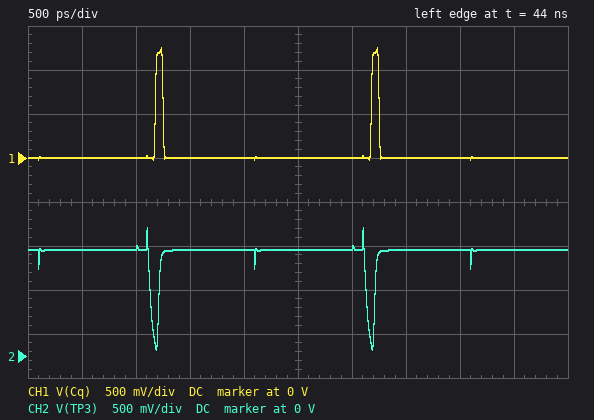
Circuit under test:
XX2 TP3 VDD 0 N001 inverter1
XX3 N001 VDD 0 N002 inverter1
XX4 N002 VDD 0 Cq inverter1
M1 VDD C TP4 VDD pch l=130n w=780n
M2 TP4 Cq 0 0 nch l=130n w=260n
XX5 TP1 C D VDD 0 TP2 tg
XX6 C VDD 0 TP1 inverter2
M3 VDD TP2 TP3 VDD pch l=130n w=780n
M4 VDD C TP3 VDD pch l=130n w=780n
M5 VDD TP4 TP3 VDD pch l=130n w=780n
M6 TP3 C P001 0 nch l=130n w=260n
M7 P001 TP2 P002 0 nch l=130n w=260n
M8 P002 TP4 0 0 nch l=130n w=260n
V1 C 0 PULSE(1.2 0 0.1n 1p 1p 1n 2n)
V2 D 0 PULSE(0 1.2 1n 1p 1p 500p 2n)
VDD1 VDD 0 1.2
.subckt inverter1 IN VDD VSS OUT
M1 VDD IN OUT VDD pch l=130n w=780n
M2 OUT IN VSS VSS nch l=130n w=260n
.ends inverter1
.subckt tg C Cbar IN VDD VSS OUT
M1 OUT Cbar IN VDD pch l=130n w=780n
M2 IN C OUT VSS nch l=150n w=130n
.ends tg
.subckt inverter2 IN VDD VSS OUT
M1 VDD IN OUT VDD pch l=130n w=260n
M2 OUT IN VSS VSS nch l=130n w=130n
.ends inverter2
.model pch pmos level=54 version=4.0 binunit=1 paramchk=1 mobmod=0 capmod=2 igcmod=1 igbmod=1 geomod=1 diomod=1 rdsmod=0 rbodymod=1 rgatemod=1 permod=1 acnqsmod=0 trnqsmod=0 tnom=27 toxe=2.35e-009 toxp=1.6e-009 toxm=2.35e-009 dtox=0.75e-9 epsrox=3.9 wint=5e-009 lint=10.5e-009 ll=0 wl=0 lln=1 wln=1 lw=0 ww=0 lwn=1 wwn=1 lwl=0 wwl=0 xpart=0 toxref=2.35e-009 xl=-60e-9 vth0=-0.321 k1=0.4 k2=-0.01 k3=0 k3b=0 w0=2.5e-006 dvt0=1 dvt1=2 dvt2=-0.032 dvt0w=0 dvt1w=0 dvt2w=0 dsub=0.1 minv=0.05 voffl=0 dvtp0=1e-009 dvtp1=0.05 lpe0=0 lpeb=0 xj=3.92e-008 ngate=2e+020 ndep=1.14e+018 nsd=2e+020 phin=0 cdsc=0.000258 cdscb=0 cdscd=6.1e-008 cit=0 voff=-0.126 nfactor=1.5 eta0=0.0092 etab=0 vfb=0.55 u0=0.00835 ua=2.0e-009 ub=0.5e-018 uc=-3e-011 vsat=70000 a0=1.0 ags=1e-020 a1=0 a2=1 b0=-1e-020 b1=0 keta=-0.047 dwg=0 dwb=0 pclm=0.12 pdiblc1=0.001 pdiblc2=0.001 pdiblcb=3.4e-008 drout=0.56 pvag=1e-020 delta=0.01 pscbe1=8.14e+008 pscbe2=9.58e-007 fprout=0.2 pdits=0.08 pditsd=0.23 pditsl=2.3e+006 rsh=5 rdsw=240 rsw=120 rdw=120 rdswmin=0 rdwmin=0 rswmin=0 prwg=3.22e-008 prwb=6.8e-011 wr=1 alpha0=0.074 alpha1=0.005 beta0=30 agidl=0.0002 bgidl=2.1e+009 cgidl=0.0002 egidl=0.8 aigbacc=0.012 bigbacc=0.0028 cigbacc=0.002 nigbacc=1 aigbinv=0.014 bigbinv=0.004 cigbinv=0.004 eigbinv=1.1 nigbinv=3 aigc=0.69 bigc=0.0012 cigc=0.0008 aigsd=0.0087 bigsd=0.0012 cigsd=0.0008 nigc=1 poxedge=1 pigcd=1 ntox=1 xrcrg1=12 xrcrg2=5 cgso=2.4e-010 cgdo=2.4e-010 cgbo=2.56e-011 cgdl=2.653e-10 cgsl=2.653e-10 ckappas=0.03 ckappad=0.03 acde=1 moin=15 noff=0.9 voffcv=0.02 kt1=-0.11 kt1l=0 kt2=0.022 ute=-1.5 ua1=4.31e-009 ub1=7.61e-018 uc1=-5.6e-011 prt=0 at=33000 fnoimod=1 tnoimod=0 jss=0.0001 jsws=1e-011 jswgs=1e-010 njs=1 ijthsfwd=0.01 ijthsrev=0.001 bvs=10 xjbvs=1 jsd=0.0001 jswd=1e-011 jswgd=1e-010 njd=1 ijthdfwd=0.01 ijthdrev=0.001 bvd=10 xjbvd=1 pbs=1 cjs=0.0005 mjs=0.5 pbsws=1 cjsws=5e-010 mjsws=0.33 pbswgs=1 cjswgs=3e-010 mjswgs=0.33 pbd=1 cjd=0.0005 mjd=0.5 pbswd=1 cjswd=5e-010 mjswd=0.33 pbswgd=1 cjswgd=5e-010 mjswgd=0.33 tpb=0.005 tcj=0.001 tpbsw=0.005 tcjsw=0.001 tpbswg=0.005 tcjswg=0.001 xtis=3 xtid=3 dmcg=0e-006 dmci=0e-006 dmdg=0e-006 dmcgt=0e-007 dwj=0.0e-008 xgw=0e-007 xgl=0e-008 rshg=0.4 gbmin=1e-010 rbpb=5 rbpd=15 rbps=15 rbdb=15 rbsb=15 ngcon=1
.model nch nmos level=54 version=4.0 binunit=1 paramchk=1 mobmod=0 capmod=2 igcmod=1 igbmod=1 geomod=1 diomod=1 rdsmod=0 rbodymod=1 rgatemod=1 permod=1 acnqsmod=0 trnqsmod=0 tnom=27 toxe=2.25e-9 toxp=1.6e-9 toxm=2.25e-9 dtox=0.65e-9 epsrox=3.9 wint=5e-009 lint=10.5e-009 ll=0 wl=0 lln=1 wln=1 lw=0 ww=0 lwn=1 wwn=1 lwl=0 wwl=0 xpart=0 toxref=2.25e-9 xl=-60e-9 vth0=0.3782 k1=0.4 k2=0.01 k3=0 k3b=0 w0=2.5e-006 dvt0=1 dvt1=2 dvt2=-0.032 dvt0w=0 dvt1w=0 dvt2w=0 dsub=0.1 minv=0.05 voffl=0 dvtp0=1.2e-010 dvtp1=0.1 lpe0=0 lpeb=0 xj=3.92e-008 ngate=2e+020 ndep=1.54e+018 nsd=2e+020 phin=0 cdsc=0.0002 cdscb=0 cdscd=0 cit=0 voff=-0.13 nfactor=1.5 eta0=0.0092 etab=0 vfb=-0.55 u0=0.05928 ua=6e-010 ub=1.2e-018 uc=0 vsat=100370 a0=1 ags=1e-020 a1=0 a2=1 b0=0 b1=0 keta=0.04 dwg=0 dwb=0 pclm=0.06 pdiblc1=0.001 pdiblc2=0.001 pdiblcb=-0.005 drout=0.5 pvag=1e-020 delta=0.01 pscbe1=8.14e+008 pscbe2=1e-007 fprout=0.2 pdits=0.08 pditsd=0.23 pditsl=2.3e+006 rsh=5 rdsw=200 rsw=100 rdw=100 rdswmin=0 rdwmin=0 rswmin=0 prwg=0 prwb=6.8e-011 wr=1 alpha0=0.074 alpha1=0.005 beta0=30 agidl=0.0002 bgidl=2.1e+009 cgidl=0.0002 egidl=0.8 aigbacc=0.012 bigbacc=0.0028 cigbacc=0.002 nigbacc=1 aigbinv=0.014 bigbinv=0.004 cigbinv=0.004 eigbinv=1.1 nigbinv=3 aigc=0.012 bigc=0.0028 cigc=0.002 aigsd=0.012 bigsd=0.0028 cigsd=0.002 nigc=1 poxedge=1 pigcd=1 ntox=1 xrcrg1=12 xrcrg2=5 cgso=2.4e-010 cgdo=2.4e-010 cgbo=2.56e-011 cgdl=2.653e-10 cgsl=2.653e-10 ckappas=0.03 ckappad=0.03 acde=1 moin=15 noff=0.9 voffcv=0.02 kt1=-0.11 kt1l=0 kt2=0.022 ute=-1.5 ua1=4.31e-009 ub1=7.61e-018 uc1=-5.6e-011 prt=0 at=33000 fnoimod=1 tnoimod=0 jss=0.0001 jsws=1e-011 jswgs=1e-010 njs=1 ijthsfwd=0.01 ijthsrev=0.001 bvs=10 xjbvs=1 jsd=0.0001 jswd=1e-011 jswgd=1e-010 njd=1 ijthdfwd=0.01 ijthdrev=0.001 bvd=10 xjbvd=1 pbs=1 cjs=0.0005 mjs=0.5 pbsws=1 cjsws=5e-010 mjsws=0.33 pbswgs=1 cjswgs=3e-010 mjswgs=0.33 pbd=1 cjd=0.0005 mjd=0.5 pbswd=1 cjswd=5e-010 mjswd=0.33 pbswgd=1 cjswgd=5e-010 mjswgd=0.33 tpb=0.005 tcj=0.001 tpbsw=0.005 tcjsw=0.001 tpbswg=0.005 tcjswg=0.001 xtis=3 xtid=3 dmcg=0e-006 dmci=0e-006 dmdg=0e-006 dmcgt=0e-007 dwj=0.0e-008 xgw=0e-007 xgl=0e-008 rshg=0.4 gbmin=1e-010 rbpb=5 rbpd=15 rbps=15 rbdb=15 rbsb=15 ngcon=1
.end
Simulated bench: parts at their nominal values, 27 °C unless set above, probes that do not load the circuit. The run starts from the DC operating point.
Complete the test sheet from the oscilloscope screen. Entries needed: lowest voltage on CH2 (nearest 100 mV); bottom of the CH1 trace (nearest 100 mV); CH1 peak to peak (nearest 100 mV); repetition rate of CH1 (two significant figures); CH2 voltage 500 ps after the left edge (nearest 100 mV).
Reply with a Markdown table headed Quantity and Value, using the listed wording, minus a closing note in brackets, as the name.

| Quantity | Value |
|---|---|
| lowest voltage on CH2 | 100 mV |
| bottom of the CH1 trace | 0 V |
| CH1 peak to peak | 1.3 V |
| repetition rate of CH1 | 500 MHz |
| CH2 voltage 500 ps after the left edge | 1.2 V |
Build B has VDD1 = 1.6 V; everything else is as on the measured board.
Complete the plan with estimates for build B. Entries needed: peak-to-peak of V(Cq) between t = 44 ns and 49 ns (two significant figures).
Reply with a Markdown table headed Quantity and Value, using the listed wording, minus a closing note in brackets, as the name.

| Quantity | Value |
|---|---|
| peak-to-peak of V(Cq) between t = 44 ns and 49 ns | 1.7 V |
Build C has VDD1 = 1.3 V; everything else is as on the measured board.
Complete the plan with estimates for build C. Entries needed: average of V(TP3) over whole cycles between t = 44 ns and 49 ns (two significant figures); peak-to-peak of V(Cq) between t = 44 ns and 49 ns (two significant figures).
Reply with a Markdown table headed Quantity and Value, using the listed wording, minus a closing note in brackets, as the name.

| Quantity | Value |
|---|---|
| average of V(TP3) over whole cycles between t = 44 ns and 49 ns | 1.3 V |
| peak-to-peak of V(Cq) between t = 44 ns and 49 ns | 1.4 V |
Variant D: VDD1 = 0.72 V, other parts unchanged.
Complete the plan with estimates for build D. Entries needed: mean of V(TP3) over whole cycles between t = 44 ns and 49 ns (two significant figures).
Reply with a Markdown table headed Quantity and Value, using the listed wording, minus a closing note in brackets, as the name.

| Quantity | Value |
|---|---|
| mean of V(TP3) over whole cycles between t = 44 ns and 49 ns | 670 mV |
